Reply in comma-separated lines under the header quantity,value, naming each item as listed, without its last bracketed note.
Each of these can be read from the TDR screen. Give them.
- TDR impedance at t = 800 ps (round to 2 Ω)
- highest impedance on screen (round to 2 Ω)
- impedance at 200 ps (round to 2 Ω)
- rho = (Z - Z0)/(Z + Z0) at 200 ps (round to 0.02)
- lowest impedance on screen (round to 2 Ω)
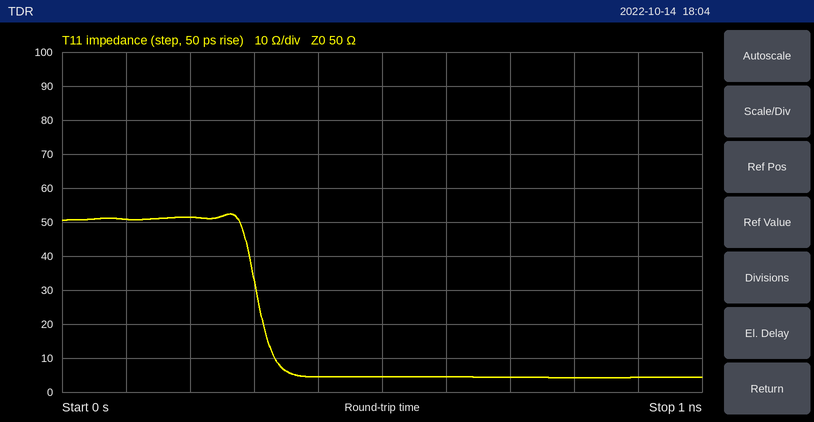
quantity,value
TDR impedance at t = 800 ps,4 Ω
highest impedance on screen,52 Ω
impedance at 200 ps,52 Ω
rho = (Z - Z0)/(Z + Z0) at 200 ps,+0.02
lowest impedance on screen,4 Ω
